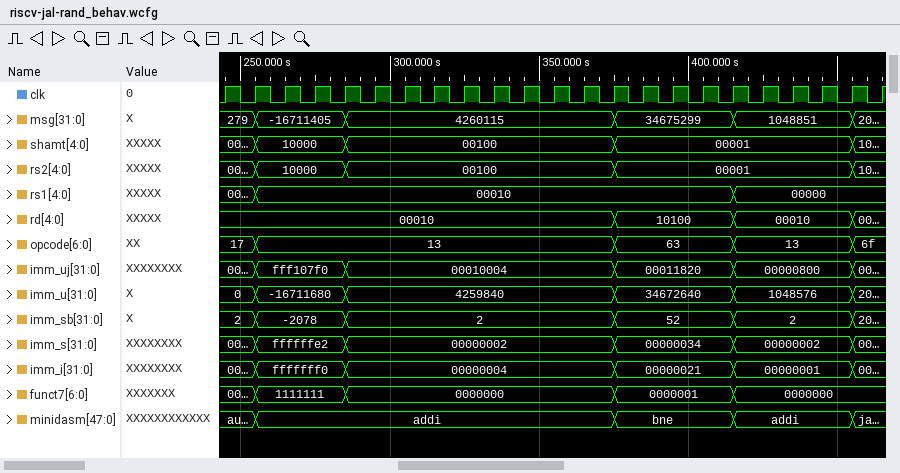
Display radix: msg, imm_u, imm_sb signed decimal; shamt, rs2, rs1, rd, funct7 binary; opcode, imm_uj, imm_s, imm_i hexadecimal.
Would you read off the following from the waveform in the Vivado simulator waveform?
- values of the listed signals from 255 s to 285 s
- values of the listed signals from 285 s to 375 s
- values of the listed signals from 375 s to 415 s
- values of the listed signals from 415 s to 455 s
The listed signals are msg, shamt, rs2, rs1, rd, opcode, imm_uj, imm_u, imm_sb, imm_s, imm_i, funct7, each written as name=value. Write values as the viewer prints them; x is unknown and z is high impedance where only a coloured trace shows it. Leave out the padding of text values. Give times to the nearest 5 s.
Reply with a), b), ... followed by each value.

a) msg=-16711405, shamt=10000, rs2=10000, rs1=00010, rd=00010, opcode=13, imm_uj=fff107f0, imm_u=-16711680, imm_sb=-2078, imm_s=ffffffe2, imm_i=fffffff0, funct7=1111111
b) msg=4260115, shamt=00100, rs2=00100, rs1=00010, rd=00010, opcode=13, imm_uj=00010004, imm_u=4259840, imm_sb=2, imm_s=00000002, imm_i=00000004, funct7=0000000
c) msg=34675299, shamt=00001, rs2=00001, rs1=00010, rd=10100, opcode=63, imm_uj=00011820, imm_u=34672640, imm_sb=52, imm_s=00000034, imm_i=00000021, funct7=0000001
d) msg=1048851, shamt=00001, rs2=00001, rs1=00000, rd=00010, opcode=13, imm_uj=00000800, imm_u=1048576, imm_sb=2, imm_s=00000002, imm_i=00000001, funct7=0000000
